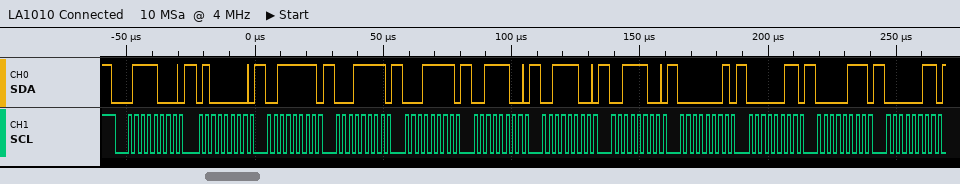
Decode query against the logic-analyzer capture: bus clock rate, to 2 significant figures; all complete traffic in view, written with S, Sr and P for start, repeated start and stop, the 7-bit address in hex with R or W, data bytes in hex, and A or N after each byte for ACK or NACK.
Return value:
400 kHz
S 3CW A 40 A 3F A 1F A 1F A 3C A 3C A 3C A 01 A 03 A 07 A 03 A
